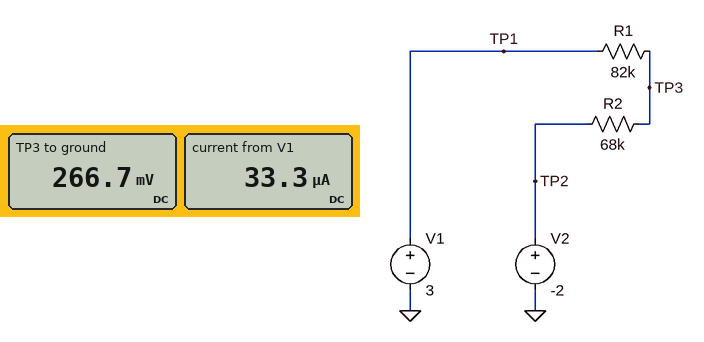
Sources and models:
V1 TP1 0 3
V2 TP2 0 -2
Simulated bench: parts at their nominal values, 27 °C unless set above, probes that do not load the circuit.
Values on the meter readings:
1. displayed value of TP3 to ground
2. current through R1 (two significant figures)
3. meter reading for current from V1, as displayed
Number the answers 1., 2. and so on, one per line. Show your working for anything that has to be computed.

1. 266.7 mV
2. (3 V - 266.7 mV) / 82 kΩ = 33 µA
3. 33.3 µA
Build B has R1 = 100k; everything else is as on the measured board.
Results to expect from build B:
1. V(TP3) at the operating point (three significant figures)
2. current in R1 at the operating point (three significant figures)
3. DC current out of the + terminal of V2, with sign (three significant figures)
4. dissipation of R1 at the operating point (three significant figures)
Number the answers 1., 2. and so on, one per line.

1. 23.8 mV
2. 29.8 µA
3. -29.8 µA
4. 88.6 µW
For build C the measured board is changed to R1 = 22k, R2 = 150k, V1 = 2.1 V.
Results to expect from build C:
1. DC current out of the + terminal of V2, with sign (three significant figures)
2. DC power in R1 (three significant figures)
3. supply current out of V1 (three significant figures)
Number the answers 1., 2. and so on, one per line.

1. -23.8 µA
2. 12.5 µW
3. 23.8 µA
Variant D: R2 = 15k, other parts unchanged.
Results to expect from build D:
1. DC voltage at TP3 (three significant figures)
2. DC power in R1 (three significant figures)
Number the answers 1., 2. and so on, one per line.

1. -1.23 V
2. 218 µW
